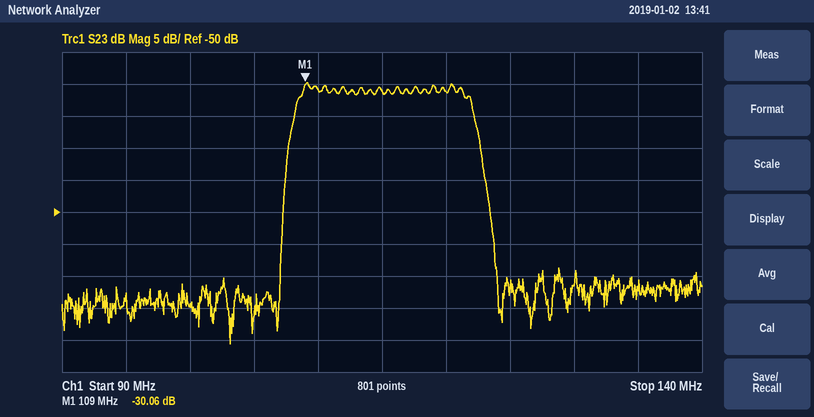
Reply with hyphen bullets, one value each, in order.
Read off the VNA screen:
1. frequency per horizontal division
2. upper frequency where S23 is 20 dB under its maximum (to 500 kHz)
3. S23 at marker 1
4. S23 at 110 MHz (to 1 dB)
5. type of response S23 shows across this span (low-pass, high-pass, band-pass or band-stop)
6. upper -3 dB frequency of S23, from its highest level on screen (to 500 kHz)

- 5 MHz
- 123.5 MHz
- -30.06 dB
- -31 dB
- band-pass
- 122.0 MHz
